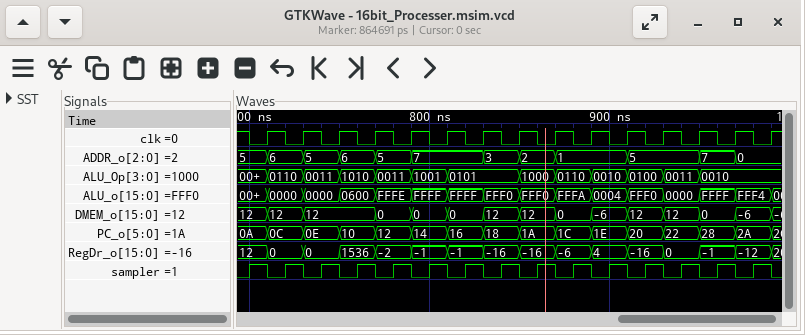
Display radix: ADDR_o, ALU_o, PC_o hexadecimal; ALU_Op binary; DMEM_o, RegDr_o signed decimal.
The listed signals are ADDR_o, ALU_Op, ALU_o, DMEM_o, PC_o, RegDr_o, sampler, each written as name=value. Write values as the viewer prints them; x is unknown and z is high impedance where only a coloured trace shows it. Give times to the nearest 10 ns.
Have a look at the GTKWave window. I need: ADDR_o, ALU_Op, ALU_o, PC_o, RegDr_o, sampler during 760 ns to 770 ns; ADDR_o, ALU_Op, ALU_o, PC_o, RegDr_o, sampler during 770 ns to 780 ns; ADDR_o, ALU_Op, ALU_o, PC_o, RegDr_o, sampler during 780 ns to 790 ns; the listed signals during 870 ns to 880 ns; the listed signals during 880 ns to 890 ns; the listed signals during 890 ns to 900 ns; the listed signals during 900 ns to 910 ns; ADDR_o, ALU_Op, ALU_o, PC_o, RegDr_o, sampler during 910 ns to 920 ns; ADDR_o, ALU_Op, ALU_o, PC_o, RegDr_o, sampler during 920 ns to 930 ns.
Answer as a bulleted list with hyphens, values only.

- ADDR_o=6, ALU_Op=1010, ALU_o=0600, PC_o=10, RegDr_o=1536, sampler=1
- ADDR_o=5, ALU_Op=0011, ALU_o=FFFE, PC_o=12, RegDr_o=-2, sampler=0
- ADDR_o=5, ALU_Op=0011, ALU_o=FFFE, PC_o=12, RegDr_o=-2, sampler=1
- ADDR_o=1, ALU_Op=0110, ALU_o=FFFA, DMEM_o=0, PC_o=1C, RegDr_o=-6, sampler=0
- ADDR_o=1, ALU_Op=0110, ALU_o=FFFA, DMEM_o=0, PC_o=1C, RegDr_o=-6, sampler=1
- ADDR_o=1, ALU_Op=0010, ALU_o=0004, DMEM_o=-6, PC_o=1E, RegDr_o=4, sampler=0
- ADDR_o=1, ALU_Op=0010, ALU_o=0004, DMEM_o=-6, PC_o=1E, RegDr_o=4, sampler=1
- ADDR_o=5, ALU_Op=0100, ALU_o=FFF0, PC_o=20, RegDr_o=-16, sampler=0
- ADDR_o=5, ALU_Op=0100, ALU_o=FFF0, PC_o=20, RegDr_o=-16, sampler=1
